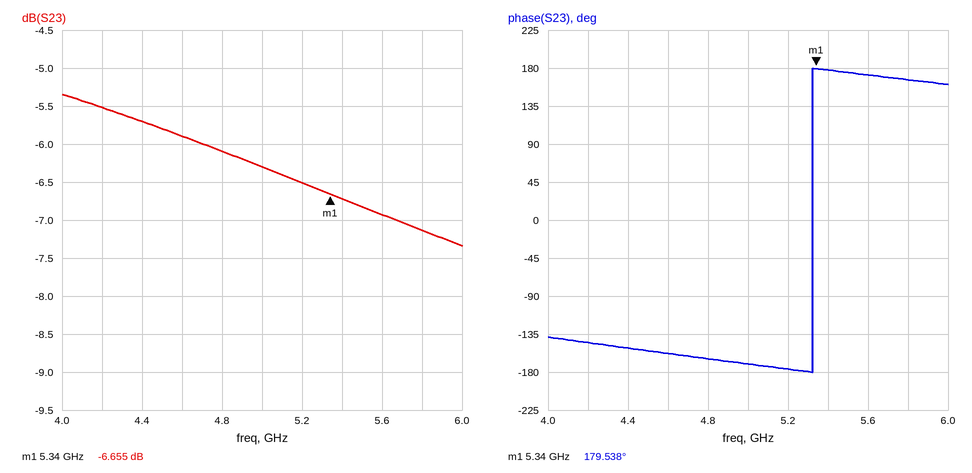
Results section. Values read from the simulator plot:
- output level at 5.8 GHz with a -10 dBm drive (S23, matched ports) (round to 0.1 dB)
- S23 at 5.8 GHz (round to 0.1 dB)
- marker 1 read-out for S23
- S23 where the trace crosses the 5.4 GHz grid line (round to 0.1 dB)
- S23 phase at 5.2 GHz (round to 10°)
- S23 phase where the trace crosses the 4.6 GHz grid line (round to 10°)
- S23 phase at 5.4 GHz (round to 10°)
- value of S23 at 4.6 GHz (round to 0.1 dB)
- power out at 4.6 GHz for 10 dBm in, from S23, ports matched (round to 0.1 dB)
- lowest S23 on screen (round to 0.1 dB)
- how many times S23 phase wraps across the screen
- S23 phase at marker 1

-17.1 dBm
-7.1 dB
-6.655 dB
-6.7 dB
-180°
-160°
180°
-5.9 dB
4.1 dBm
-7.3 dB
1
179.538°
